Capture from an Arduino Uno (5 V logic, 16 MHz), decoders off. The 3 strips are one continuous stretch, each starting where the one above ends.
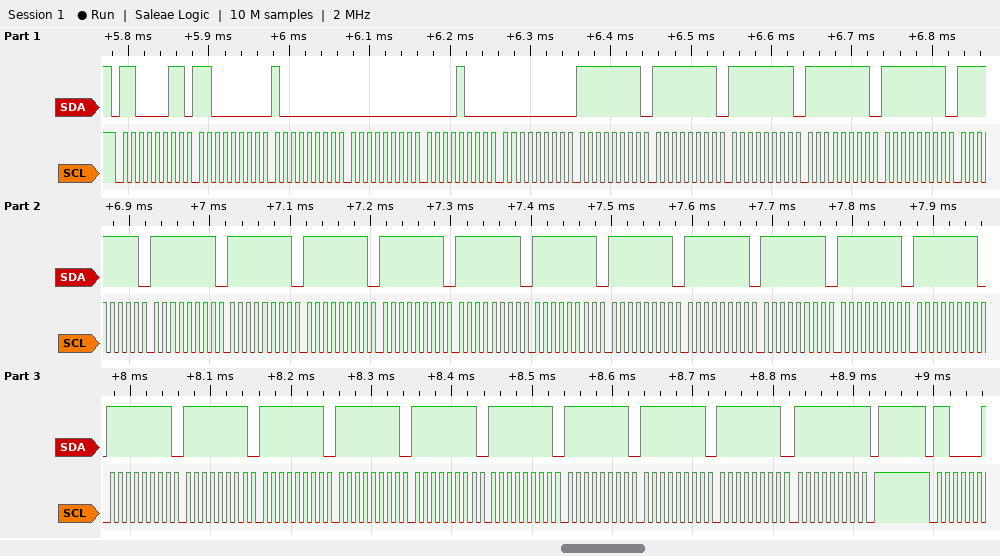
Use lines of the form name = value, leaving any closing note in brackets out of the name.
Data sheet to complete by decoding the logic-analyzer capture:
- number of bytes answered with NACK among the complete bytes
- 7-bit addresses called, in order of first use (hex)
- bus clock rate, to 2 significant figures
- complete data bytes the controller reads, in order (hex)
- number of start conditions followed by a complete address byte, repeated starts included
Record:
number of bytes answered with NACK among the complete bytes = 1
7-bit addresses called, in order of first use = 0x61
bus clock rate, to 2 significant figures = 100 kHz
complete data bytes the controller reads, in order = C0 80 00 08 00 FF FF FF FF FF FF FF FF FF FF FF FF FF FF FF FF FF FF FF FF FF FF FF FF FF FF FF
number of start conditions followed by a complete address byte, repeated starts included = 1
